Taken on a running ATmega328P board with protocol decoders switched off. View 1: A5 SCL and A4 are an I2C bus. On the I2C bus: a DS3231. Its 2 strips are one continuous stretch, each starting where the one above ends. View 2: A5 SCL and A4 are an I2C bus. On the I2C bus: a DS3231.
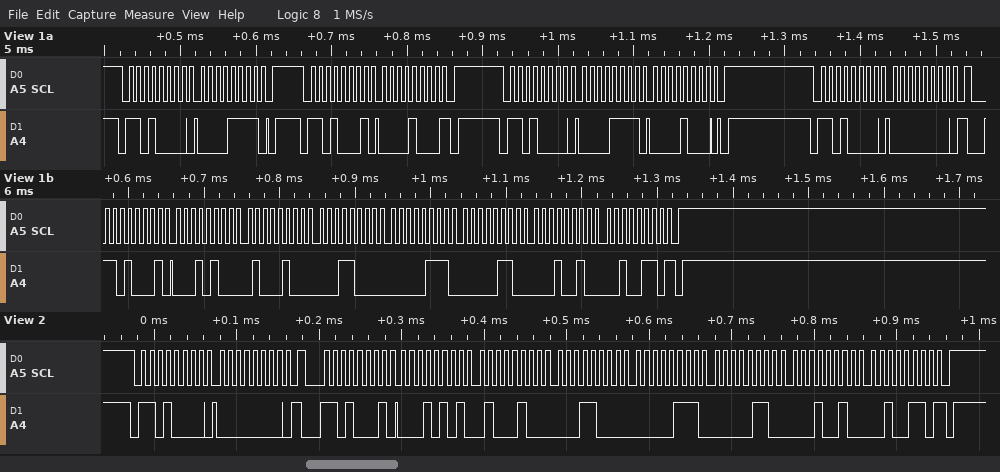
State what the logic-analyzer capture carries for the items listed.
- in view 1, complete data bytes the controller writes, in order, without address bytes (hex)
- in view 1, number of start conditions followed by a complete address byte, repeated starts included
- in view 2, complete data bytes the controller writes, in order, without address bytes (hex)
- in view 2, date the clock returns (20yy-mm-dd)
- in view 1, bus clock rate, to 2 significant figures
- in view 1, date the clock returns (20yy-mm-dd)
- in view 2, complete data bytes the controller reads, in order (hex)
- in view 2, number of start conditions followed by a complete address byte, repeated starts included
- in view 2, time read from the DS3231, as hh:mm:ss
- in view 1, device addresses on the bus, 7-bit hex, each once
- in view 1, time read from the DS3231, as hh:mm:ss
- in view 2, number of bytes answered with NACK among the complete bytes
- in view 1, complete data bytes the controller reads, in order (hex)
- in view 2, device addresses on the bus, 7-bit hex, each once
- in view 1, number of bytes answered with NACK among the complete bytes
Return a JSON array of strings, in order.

["0F 0F 08 00", "5", "00", "2026-12-06", "100 kHz", "2026-12-06", "15 44 18 07 06 12 26", "2", "18:44:15", "0x68", "18:44:14", "1", "08 14 44 18 07 06 12 26", "0x68", "2"]
